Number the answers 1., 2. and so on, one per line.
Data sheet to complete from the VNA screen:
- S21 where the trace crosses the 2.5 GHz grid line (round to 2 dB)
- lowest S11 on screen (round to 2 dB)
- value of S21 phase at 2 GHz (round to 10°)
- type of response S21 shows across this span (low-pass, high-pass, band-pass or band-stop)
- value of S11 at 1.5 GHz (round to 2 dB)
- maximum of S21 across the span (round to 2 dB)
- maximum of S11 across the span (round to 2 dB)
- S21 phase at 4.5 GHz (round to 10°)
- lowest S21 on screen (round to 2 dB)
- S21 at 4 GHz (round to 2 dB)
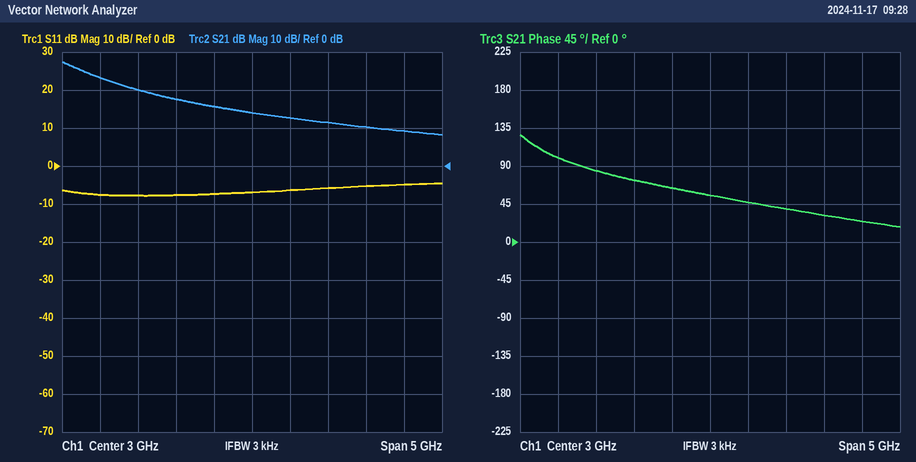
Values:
1. 16 dB
2. -8 dB
3. 70°
4. low-pass
5. -8 dB
6. 28 dB
7. -4 dB
8. 30°
9. 8 dB
10. 12 dB
